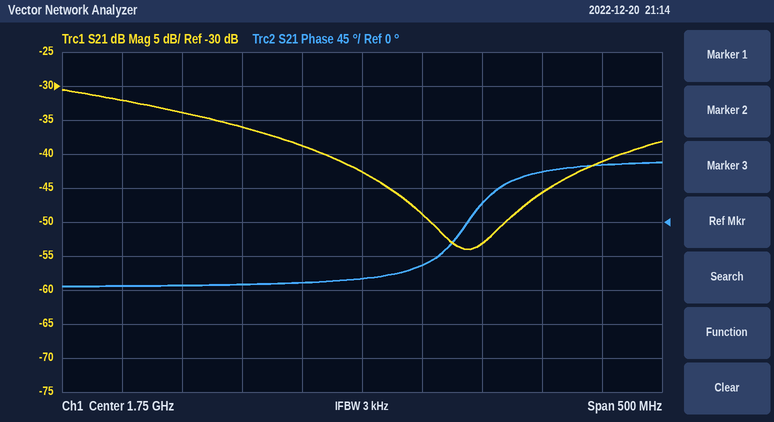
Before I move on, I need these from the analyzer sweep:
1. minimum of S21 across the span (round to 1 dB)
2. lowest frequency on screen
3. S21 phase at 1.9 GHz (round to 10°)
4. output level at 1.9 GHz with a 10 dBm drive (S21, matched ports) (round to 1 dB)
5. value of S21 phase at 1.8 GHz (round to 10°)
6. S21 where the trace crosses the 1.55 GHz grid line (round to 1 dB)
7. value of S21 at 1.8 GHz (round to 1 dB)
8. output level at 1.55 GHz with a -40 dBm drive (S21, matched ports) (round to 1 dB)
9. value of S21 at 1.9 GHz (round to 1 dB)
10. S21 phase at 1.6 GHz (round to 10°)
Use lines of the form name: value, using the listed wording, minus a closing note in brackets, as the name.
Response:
minimum of S21 across the span: -54 dB
lowest frequency on screen: 1.5 GHz
S21 phase at 1.9 GHz: 70°
output level at 1.9 GHz with a 10 dBm drive (S21, matched ports): -36 dBm
value of S21 phase at 1.8 GHz: -60°
S21 where the trace crosses the 1.55 GHz grid line: -32 dB
value of S21 at 1.8 GHz: -49 dB
output level at 1.55 GHz with a -40 dBm drive (S21, matched ports): -72 dBm
value of S21 at 1.9 GHz: -46 dB
S21 phase at 1.6 GHz: -80°
